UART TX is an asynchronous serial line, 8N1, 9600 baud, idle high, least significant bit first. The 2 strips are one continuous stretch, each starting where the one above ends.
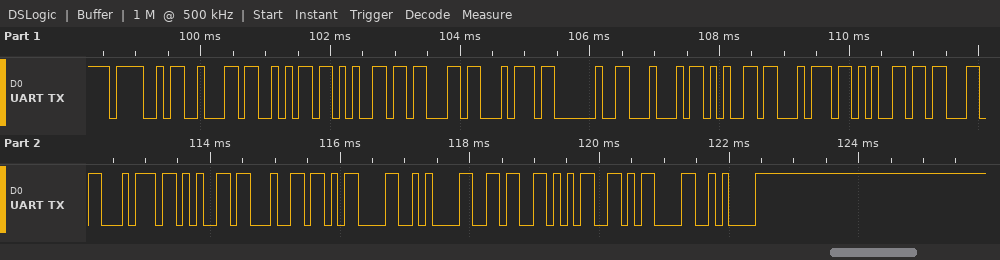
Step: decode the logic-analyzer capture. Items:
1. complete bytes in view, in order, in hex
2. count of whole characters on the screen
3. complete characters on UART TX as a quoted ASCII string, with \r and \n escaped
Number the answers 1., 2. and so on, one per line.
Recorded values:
1. 4F 62 6A 65 63 74 20 44 65 74 65 63 74 65 64 0D 0A 36 35 0D 0A
2. 21
3. "Object Detected\r\n65\r\n"
